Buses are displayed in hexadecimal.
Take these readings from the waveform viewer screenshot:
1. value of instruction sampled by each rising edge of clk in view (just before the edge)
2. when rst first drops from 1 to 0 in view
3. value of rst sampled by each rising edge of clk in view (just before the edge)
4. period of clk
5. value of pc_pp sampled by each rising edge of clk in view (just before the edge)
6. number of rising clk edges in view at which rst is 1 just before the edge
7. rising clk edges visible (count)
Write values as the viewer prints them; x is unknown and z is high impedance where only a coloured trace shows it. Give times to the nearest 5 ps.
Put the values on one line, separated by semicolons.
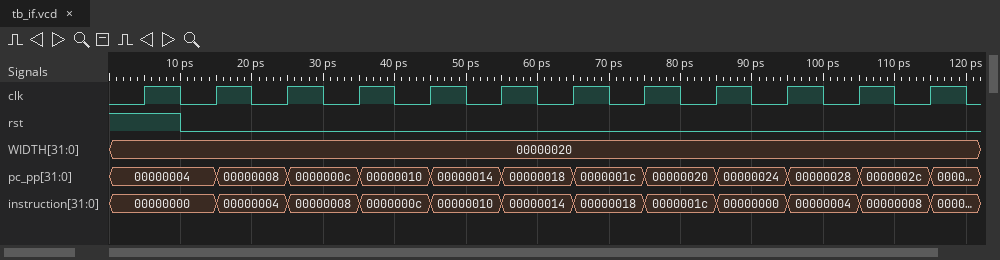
00000000, 00000000, 00000004, 00000008, 0000000c, 00000010, 00000014, 00000018, 0000001c, 00000000, 00000004, 00000008; 10 ps; 1 0 0 0 0 0 0 0 0 0 0 0; 10 ps; 00000004, 00000004, 00000008, 0000000c, 00000010, 00000014, 00000018, 0000001c, 00000020, 00000024, 00000028, 0000002c; 1; 12
